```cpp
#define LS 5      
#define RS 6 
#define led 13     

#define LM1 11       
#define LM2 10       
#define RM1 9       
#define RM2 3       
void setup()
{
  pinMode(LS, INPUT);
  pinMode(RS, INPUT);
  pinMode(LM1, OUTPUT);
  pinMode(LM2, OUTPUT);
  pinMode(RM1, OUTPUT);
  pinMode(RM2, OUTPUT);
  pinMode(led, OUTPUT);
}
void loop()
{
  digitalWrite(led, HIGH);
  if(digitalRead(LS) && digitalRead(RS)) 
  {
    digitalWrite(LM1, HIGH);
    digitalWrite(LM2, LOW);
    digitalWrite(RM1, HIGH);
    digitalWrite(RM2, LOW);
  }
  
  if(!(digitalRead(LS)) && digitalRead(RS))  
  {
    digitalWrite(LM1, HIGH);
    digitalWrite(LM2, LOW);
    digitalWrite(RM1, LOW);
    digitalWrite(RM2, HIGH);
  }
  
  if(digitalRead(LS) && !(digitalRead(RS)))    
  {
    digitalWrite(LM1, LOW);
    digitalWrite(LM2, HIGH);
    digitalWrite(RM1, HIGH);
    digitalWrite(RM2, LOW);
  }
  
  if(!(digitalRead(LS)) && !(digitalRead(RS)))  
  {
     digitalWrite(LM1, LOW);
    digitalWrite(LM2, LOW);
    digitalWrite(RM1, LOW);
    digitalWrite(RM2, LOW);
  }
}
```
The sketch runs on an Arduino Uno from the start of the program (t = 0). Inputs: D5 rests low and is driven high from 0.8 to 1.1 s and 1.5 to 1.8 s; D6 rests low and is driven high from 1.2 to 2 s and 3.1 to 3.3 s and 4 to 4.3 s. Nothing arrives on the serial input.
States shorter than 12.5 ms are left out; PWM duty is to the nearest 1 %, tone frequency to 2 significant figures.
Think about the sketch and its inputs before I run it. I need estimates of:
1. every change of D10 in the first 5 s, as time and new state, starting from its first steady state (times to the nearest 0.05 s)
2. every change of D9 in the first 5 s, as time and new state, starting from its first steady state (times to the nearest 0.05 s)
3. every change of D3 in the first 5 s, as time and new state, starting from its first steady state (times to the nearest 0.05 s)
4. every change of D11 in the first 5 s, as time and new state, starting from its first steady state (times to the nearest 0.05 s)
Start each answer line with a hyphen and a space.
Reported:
- 0 s low; 0.8 s high; 1.1 s low
- 0 s low; 0.8 s high; 1.1 s low; 1.5 s high; 1.8 s low
- 0 s low; 1.2 s high; 1.5 s low; 1.8 s high; 2 s low; 3.1 s high; 3.3 s low; 4 s high; 4.3 s low
- 0 s low; 1.2 s high; 2 s low; 3.1 s high; 3.3 s low; 4 s high; 4.3 s low
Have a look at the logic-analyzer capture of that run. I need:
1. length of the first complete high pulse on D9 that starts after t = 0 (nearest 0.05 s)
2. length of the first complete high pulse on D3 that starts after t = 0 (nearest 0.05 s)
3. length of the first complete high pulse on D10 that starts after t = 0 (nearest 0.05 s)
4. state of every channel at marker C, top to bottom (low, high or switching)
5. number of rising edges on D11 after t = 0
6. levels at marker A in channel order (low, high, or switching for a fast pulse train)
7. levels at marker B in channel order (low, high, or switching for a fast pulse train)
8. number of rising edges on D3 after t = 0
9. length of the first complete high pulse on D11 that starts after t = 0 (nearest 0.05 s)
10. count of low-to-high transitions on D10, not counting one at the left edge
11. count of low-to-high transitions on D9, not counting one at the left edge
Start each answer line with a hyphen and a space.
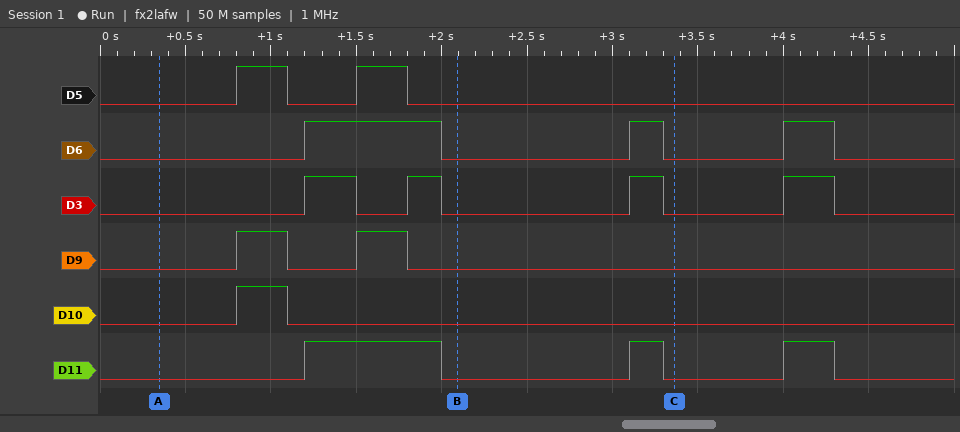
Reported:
- 0.30 s
- 0.30 s
- 0.30 s
- D5 low, D6 low, D3 low, D9 low, D10 low, D11 low
- 3
- D5 low, D6 low, D3 low, D9 low, D10 low, D11 low
- D5 low, D6 low, D3 low, D9 low, D10 low, D11 low
- 4
- 0.80 s
- 1
- 2
